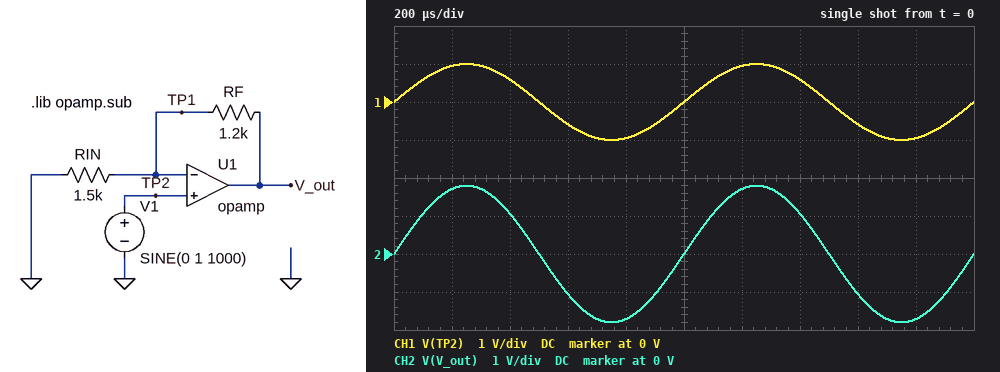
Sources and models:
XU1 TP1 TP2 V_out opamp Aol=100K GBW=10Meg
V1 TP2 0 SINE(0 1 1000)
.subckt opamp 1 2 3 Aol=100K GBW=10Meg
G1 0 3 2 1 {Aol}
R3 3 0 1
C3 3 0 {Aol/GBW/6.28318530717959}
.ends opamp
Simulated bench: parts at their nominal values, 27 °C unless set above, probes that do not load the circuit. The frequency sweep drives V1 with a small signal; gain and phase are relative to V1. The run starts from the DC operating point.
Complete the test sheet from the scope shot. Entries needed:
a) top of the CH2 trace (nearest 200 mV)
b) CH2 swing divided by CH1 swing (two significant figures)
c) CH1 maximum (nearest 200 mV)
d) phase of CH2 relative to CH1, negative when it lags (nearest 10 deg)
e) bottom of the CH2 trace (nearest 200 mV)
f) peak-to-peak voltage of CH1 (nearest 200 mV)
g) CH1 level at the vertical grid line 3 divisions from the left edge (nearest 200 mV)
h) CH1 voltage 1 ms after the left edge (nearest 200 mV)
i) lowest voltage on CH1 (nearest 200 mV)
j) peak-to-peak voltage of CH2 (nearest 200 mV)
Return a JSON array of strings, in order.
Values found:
["1.8 V", "1.8", "1.0 V", "0 deg", "-1.8 V", "2.0 V", "-600 mV", "0 V", "-1.0 V", "3.6 V"]
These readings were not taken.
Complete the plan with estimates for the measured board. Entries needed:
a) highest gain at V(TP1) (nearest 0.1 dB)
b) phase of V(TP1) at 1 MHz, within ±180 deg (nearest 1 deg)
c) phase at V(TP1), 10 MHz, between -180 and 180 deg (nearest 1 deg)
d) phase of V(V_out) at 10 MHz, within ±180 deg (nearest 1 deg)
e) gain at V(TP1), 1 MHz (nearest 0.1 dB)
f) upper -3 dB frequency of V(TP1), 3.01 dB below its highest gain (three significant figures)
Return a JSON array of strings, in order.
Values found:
["0 dB", "-10 deg", "-61 deg", "-61 deg", "-0.1 dB", "5.56 MHz"]
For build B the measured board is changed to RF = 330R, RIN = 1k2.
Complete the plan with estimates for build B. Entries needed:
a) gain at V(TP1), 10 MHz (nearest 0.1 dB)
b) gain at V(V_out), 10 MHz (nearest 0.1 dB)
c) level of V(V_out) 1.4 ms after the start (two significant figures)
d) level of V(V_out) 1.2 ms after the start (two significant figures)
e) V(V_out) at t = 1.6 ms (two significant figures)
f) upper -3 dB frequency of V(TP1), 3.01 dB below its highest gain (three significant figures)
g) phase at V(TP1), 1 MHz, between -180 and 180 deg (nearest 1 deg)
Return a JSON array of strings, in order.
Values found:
["-4.2 dB", "-2.1 dB", "750 mV", "1.2 V", "-750 mV", "7.84 MHz", "-7 deg"]
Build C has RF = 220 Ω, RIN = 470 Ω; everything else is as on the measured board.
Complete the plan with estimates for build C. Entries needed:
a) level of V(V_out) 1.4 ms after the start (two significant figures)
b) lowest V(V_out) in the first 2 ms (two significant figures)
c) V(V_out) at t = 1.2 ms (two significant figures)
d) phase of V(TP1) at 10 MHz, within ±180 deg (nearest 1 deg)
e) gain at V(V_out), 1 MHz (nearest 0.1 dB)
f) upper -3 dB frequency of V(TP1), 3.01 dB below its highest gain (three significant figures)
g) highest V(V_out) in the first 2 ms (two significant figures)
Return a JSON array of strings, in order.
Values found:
["860 mV", "-1.5 V", "1.4 V", "-56 deg", "3.2 dB", "6.81 MHz", "1.5 V"]
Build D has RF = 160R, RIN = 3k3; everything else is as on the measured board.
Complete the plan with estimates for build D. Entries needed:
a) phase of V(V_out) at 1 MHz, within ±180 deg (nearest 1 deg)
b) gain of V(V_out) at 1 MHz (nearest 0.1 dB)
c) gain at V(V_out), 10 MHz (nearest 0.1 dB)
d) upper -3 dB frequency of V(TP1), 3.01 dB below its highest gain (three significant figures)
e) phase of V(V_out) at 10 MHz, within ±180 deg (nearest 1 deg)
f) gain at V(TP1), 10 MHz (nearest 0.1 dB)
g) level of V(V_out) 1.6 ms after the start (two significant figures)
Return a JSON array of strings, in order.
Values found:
["-6 deg", "0.4 dB", "-2.8 dB", "9.54 MHz", "-46 deg", "-3.2 dB", "-620 mV"]
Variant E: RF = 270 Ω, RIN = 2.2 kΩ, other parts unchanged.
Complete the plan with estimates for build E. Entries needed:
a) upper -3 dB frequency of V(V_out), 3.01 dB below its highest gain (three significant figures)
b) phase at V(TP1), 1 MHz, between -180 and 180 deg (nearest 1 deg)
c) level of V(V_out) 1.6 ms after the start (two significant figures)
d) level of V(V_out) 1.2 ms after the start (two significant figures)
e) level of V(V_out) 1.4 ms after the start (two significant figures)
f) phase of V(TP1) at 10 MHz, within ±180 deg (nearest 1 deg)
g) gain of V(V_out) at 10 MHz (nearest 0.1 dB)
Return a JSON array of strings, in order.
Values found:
["8.91 MHz", "-6 deg", "-660 mV", "1.1 V", "660 mV", "-48 deg", "-2.5 dB"]
